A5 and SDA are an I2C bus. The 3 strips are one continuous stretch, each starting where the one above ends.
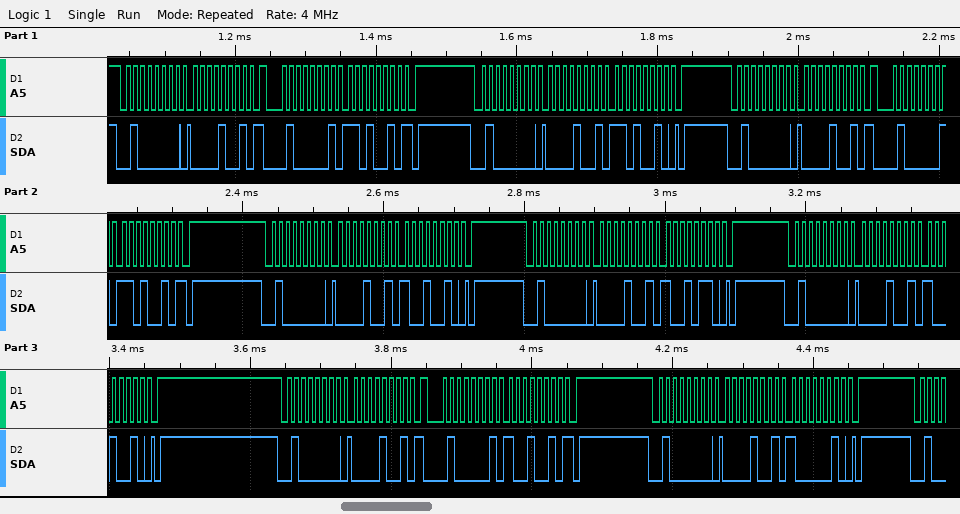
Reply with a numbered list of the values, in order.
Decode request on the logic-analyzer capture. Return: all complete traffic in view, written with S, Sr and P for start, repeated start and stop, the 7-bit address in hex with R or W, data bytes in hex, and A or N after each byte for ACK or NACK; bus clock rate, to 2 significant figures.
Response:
1. S 20W A 09 A Sr 20R A D2 N P S 20W A 09 A D2 A P S 20W A 09 A Sr 20R A D2 N P S 20W A 09 A 92 A P S 20W A 09 A 96 A P S 20W A 09 A 92 A P S 20W A 09 A Sr 20R A 92 N P S 20W A 09 A 82 A P
2. 100 kHz
